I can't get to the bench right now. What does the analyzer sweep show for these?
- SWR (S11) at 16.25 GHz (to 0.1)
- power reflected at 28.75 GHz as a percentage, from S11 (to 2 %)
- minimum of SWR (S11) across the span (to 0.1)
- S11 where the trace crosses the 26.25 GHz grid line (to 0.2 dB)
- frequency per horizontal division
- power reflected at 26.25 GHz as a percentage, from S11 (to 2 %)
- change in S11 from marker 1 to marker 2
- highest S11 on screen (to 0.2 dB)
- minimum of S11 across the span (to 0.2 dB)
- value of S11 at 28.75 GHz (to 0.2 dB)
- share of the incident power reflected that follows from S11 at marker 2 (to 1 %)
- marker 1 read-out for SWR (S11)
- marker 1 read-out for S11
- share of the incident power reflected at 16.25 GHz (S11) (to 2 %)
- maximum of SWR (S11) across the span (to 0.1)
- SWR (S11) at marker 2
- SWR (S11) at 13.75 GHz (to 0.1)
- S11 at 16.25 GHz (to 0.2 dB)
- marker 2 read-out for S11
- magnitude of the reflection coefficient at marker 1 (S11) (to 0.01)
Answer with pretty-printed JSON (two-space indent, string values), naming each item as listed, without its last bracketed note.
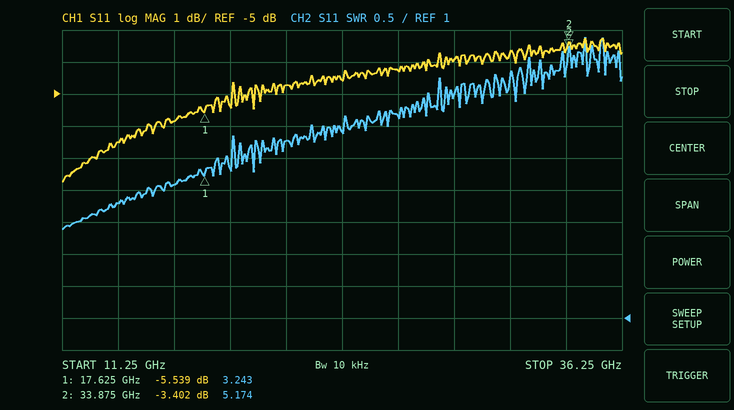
{
  "SWR (S11) at 16.25 GHz": "3.1",
  "power reflected at 28.75 GHz as a percentage, from S11": "40 %",
  "minimum of SWR (S11) across the span": "2.4",
  "S11 where the trace crosses the 26.25 GHz grid line": "-4.2 dB",
  "frequency per horizontal division": "2.5 GHz",
  "power reflected at 26.25 GHz as a percentage, from S11": "38 %",
  "change in S11 from marker 1 to marker 2": "2.137 dB",
  "highest S11 on screen": "-3.2 dB",
  "minimum of S11 across the span": "-7.8 dB",
  "value of S11 at 28.75 GHz": "-4.0 dB",
  "share of the incident power reflected that follows from S11 at marker 2": "46 %",
  "marker 1 read-out for SWR": "3.243",
  "marker 1 read-out for S11": "-5.539 dB",
  "share of the incident power reflected at 16.25 GHz (S11)": "26 %",
  "maximum of SWR (S11) across the span": "5.4",
  "SWR (S11) at marker 2": "5.174",
  "SWR (S11) at 13.75 GHz": "2.8",
  "S11 at 16.25 GHz": "-5.8 dB",
  "marker 2 read-out for S11": "-3.402 dB",
  "magnitude of the reflection coefficient at marker 1 (S11)": "0.53"
}
